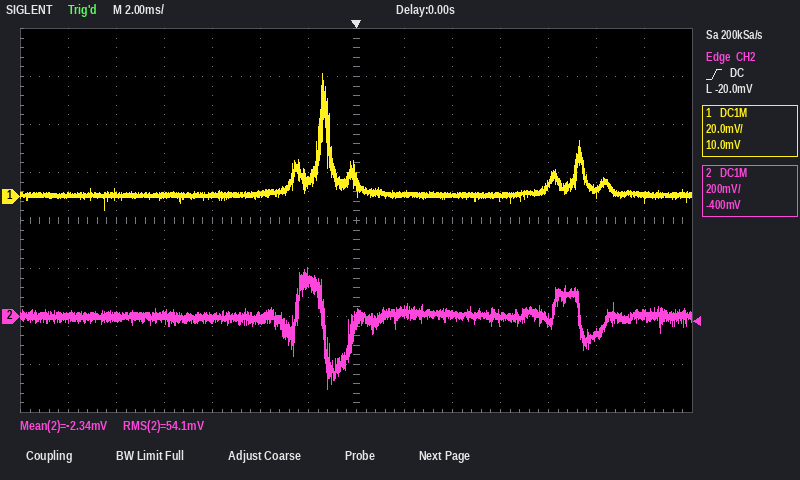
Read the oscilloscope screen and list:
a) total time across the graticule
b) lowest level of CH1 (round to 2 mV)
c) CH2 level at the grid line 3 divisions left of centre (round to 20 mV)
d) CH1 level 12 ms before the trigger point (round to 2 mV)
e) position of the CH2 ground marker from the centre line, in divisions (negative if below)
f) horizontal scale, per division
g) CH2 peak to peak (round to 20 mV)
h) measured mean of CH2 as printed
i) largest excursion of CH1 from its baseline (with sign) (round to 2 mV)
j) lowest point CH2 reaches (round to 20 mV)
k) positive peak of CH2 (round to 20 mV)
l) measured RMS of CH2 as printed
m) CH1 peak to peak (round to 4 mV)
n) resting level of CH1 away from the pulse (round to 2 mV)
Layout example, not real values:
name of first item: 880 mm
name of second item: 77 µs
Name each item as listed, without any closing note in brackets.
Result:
total time across the graticule: 28 ms
lowest level of CH1: -6 mV
CH2 level at the grid line 3 divisions left of centre: 0 mV
CH1 level 12 ms before the trigger point: 0 mV
position of the CH2 ground marker from the centre line, in divisions: -2.0 div
horizontal scale, per division: 2 ms
CH2 peak to peak: 500 mV
measured mean of CH2 as printed: -2.34 mV
largest excursion of CH1 from its baseline (with sign): +50 mV
lowest point CH2 reaches: -300 mV
positive peak of CH2: 200 mV
measured RMS of CH2 as printed: 54.1 mV
CH1 peak to peak: 56 mV
resting level of CH1 away from the pulse: 0 mV
